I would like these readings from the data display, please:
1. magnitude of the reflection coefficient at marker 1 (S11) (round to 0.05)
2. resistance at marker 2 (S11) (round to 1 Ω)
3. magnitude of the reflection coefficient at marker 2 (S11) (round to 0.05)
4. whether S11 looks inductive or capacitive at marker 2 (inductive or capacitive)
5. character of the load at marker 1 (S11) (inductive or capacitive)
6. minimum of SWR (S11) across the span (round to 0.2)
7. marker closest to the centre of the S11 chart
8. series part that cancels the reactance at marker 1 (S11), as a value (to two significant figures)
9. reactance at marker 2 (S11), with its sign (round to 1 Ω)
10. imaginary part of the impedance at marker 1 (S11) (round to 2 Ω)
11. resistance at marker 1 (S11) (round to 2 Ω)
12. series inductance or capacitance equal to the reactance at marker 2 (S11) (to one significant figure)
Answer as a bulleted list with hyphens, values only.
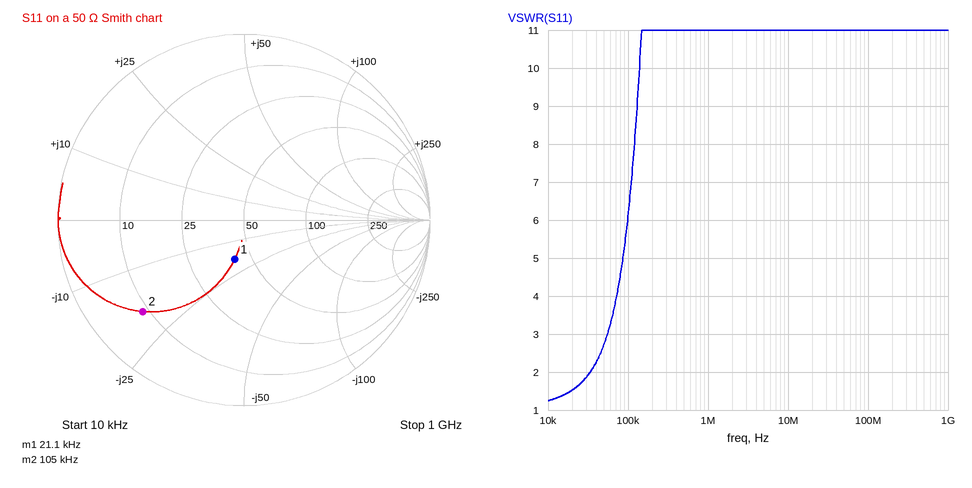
- 0.20
- 9 Ω
- 0.75
- capacitive
- capacitive
- 1.2
- marker 1
- 140 µH
- -19 Ω
- -18 Ω
- 42 Ω
- 80 nF
